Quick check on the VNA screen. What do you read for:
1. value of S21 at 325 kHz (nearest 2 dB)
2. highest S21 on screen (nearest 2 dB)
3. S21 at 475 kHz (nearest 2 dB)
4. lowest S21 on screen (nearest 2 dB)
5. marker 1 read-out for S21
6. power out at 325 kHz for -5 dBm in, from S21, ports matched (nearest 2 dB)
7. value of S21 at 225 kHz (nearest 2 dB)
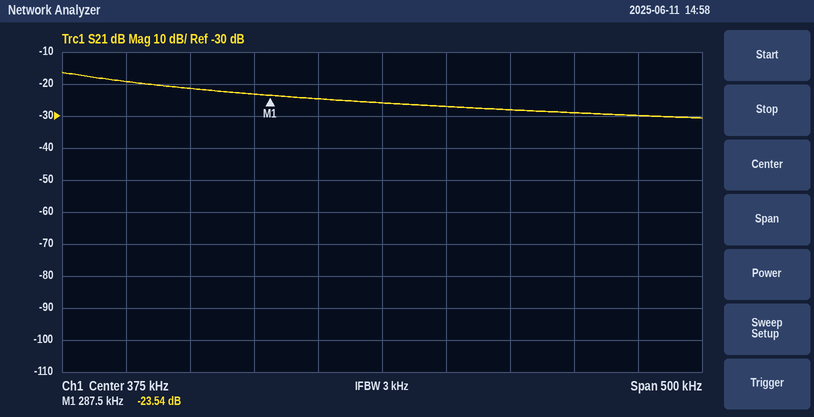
-24 dB
-16 dB
-28 dB
-30 dB
-23.54 dB
-30 dBm
-22 dB
